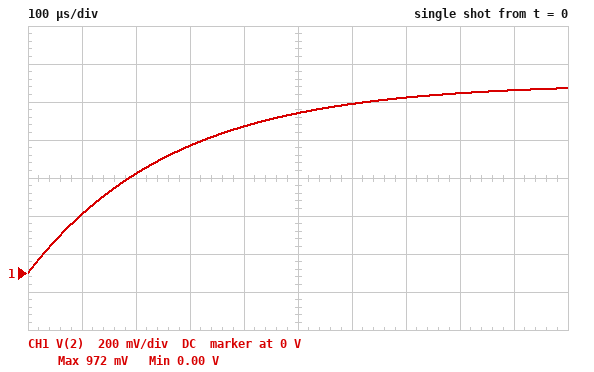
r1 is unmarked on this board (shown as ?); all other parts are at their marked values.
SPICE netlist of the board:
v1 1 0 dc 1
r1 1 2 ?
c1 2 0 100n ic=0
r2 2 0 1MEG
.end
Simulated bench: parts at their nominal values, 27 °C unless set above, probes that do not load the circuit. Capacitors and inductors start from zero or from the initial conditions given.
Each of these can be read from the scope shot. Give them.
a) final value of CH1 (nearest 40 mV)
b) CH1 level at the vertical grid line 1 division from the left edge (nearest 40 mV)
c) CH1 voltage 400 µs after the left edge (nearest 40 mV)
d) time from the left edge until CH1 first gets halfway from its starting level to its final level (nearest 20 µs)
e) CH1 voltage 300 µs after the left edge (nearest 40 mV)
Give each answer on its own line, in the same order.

960 mV
320 mV
760 mV
180 µs
680 mV
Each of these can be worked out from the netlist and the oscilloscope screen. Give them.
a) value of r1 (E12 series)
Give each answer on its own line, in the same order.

2.7 kΩ
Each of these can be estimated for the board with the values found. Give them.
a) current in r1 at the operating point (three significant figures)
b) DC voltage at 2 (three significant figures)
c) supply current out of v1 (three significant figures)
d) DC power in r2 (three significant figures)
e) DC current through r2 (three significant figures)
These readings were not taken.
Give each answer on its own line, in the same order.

997 nA
997 mV
997 nA
995 nW
997 nA
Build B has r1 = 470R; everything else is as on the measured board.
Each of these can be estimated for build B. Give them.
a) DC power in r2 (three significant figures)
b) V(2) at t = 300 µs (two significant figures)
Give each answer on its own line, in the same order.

999 nW
1.0 V
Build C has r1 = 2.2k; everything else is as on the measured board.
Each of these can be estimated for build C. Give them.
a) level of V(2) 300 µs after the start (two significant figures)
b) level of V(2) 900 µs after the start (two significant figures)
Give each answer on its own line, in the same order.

740 mV
980 mV
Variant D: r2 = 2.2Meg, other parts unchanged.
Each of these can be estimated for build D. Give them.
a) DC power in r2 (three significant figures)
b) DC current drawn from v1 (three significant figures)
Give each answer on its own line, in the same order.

453 nW
454 nA
